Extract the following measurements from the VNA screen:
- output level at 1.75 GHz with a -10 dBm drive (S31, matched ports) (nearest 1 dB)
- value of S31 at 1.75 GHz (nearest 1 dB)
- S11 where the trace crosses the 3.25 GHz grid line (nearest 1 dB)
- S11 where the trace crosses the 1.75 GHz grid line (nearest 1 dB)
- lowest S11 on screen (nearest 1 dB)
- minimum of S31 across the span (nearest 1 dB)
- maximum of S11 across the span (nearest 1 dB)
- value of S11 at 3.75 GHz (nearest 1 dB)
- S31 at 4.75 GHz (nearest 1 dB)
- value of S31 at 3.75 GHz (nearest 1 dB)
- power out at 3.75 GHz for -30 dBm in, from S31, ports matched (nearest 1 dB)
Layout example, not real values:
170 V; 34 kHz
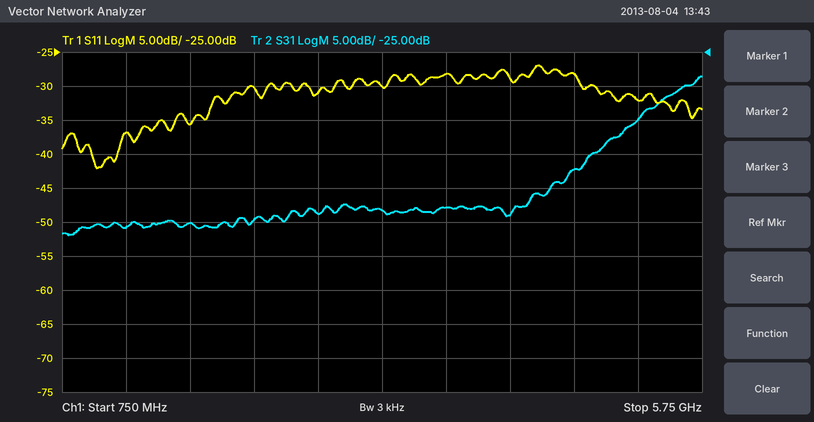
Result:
-60 dBm; -50 dB; -30 dB; -36 dB; -42 dB; -52 dB; -27 dB; -28 dB; -42 dB; -48 dB; -78 dBm
